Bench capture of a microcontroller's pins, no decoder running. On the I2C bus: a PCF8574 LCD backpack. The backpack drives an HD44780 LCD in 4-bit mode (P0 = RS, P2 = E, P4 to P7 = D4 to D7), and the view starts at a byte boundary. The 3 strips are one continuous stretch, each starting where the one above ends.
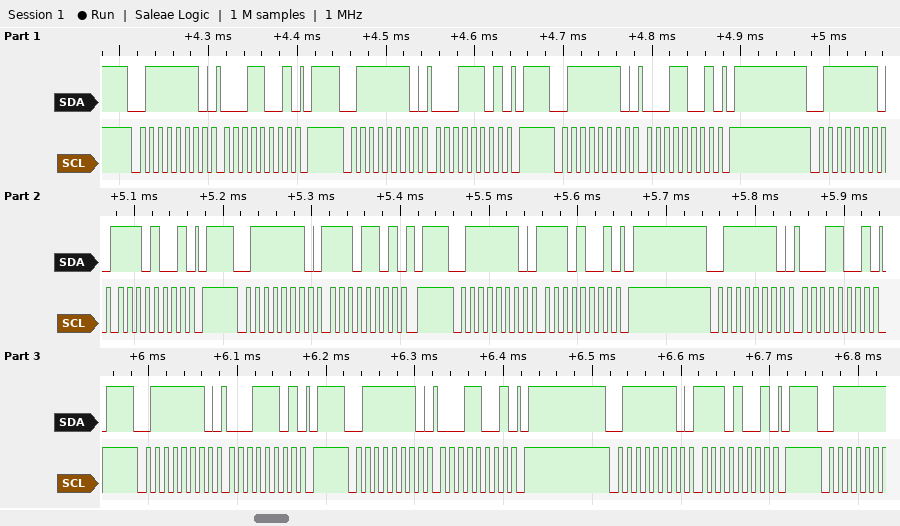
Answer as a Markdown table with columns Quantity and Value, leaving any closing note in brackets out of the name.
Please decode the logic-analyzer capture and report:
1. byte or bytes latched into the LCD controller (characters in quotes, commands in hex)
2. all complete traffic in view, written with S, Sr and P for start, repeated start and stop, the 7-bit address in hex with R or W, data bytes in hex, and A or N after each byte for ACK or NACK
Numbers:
| Quantity | Value |
|---|---|
| byte or bytes latched into the LCD controller | data 0x1E |
| all complete traffic in view, written with S, Sr and P for start, repeated start and stop, the 7-bit address in hex with R or W, data bytes in hex, and A or N after each byte for ACK or NACK | S 3FW A 19 A P S 3FW A 1D A P S 3FW A 19 A P S 3FW A E9 A P S 3FW A ED A P S 3FW A E9 A P S 3FW A 19 A P S 3FW A 1D A P S 3FW A 19 A P S 3FW A E9 A P |
